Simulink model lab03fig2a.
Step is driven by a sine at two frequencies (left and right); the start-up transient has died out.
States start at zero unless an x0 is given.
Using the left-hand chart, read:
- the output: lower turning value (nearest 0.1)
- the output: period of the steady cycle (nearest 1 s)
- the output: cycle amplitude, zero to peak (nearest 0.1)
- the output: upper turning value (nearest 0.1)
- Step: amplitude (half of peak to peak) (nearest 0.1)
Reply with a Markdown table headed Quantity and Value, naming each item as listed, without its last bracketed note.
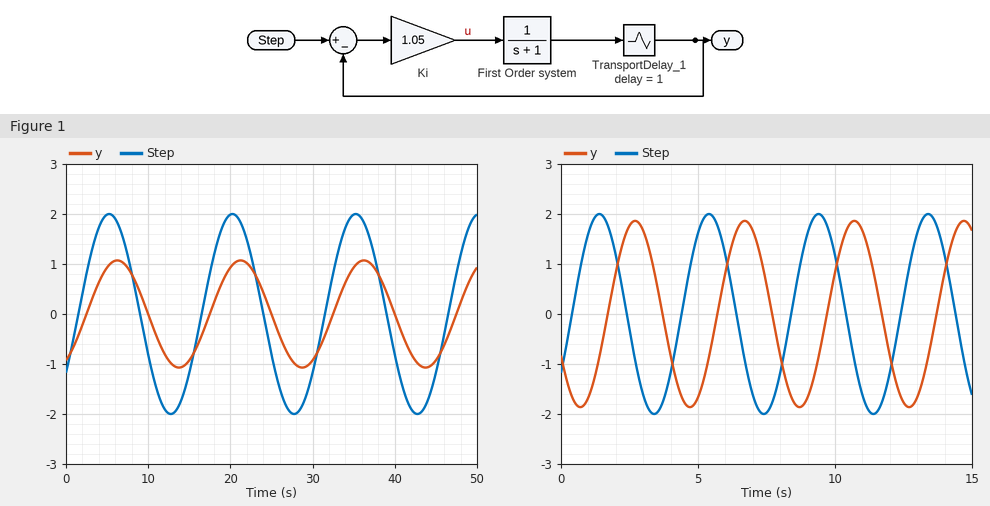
| Quantity | Value |
|---|---|
| the output: lower turning value | -1.1 |
| the output: period of the steady cycle | 15 s |
| the output: cycle amplitude, zero to peak | 1.1 |
| the output: upper turning value | 1.1 |
| Step: amplitude (half of peak to peak) | 2.0 |
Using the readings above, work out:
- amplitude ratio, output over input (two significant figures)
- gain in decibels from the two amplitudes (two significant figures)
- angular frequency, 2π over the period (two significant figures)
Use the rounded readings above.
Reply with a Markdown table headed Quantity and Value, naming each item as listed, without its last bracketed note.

| Quantity | Value |
|---|---|
| amplitude ratio, output over input | 0.55 |
| gain in decibels from the two amplitudes | -5.2 dB |
| angular frequency, 2π over the period | 0.42 rad/s |
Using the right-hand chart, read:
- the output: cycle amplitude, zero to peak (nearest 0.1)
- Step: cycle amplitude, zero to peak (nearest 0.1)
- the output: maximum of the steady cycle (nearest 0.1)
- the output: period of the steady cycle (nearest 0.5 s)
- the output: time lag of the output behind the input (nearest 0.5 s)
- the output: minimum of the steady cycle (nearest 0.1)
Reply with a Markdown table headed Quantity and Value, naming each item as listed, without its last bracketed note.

| Quantity | Value |
|---|---|
| the output: cycle amplitude, zero to peak | 1.9 |
| Step: cycle amplitude, zero to peak | 2.0 |
| the output: maximum of the steady cycle | 1.9 |
| the output: period of the steady cycle | 4.0 s |
| the output: time lag of the output behind the input | 1.5 s |
| the output: minimum of the steady cycle | -1.9 |
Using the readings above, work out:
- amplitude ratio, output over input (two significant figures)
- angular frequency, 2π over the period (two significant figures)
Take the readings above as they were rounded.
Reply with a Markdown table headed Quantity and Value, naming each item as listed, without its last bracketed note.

| Quantity | Value |
|---|---|
| amplitude ratio, output over input | 0.95 |
| angular frequency, 2π over the period | 1.6 rad/s |
